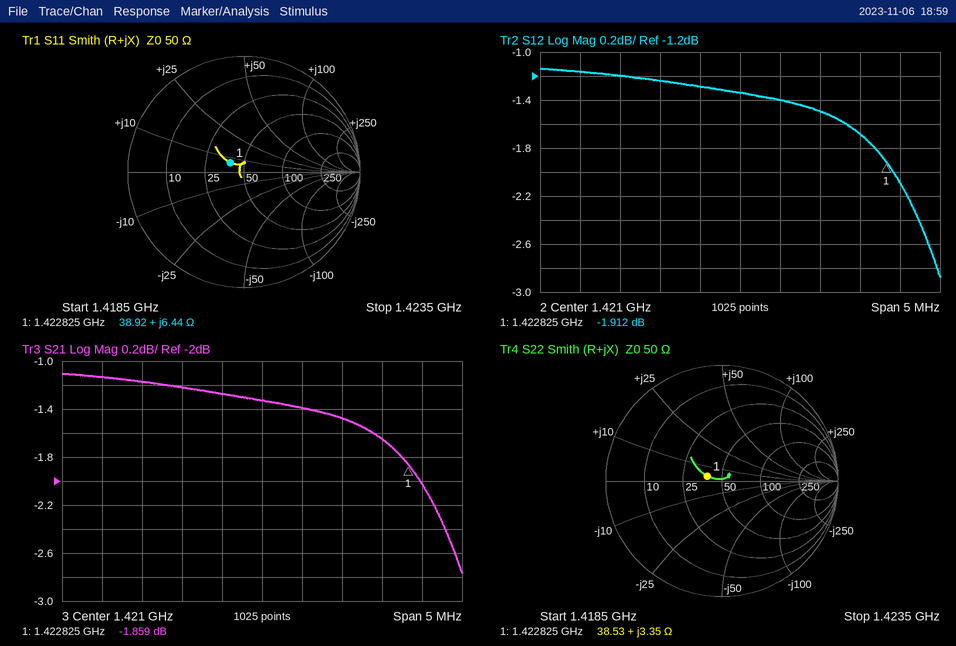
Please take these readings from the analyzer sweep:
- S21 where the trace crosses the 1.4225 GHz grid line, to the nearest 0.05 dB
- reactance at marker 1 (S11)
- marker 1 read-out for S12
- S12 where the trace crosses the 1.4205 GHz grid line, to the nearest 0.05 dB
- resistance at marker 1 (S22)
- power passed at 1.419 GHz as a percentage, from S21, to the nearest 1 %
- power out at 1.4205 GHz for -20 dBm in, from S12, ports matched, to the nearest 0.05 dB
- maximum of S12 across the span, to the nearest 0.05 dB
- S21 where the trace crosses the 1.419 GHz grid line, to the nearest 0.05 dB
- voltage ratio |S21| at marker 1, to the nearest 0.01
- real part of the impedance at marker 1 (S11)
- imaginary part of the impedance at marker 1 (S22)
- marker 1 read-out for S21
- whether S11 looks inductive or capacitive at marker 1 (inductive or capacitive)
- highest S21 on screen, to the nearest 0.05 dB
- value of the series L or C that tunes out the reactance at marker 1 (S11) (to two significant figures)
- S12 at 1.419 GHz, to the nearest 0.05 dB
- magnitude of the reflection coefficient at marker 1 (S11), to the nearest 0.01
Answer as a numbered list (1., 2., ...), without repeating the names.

1. -1.65 dB
2. +6.44 Ω
3. -1.912 dB
4. -1.30 dB
5. 38.53 Ω
6. 77 %
7. -21.30 dBm
8. -1.15 dB
9. -1.15 dB
10. 0.81
11. 38.92 Ω
12. +3.35 Ω
13. -1.859 dB
14. inductive
15. -1.10 dB
16. 17 pF
17. -1.15 dB
18. 0.14
